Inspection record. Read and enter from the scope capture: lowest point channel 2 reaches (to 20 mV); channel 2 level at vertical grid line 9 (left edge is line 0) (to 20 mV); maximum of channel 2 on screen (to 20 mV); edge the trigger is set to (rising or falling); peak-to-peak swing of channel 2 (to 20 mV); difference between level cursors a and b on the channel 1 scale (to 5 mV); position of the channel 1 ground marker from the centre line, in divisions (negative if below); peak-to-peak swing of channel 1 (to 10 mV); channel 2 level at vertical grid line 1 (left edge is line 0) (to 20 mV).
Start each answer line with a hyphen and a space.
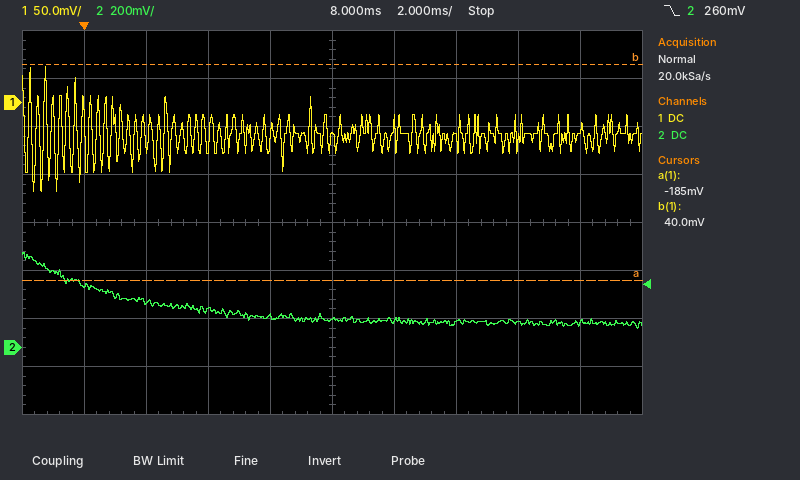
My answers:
- 80 mV
- 100 mV
- 400 mV
- falling
- 320 mV
- 225 mV
- +2.5 div
- 130 mV
- 260 mV
